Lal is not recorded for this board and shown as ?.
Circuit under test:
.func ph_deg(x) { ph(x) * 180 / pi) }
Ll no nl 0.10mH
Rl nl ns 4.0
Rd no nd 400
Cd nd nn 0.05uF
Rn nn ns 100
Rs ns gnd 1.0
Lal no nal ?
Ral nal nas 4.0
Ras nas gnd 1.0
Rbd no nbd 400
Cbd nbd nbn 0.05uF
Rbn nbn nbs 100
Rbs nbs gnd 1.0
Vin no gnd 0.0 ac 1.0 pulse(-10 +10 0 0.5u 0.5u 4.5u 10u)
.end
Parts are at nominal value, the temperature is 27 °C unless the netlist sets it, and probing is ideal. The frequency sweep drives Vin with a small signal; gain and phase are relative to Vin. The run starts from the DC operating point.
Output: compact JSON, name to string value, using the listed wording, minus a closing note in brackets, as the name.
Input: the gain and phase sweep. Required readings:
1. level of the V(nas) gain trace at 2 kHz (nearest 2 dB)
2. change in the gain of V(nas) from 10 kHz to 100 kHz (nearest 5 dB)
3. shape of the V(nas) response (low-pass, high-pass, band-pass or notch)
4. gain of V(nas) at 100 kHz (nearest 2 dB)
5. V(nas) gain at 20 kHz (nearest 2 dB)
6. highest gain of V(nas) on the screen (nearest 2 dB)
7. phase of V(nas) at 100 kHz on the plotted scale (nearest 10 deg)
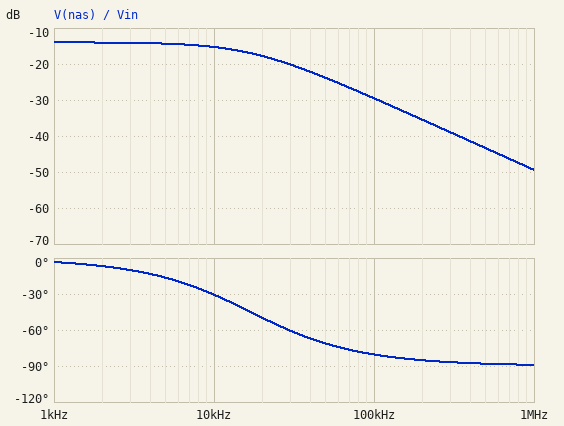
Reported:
{"level of the V(nas) gain trace at 2 kHz": "-14 dB", "change in the gain of V(nas) from 10 kHz to 100 kHz": "-15 dB", "shape of the V(nas) response": "low-pass", "gain of V(nas) at 100 kHz": "-30 dB", "V(nas) gain at 20 kHz": "-18 dB", "highest gain of V(nas) on the screen": "-14 dB", "phase of V(nas) at 100 kHz on the plotted scale": "-80 deg"}
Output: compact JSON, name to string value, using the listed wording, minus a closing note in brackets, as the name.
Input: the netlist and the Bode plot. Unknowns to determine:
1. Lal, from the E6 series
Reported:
{"Lal, from the E6 series": "47 µH"}
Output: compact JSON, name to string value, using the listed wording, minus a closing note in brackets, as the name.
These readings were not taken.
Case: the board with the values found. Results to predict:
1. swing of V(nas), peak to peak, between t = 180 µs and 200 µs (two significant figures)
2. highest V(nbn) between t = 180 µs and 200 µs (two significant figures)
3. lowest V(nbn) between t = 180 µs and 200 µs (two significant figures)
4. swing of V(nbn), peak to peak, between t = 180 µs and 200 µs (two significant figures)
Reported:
{"swing of V(nas), peak to peak, between t = 180 µs and 200 µs": "990 mV", "highest V(nbn) between t = 180 µs and 200 µs": "2.2 V", "lowest V(nbn) between t = 180 µs and 200 µs": "-2.2 V", "swing of V(nbn), peak to peak, between t = 180 µs and 200 µs": "4.4 V"}
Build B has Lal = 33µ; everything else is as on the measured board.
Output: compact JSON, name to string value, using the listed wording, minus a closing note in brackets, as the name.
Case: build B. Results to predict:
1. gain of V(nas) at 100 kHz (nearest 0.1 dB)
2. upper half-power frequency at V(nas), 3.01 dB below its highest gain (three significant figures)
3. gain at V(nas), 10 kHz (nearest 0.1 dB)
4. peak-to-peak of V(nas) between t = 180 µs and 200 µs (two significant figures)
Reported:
{"gain of V(nas) at 100 kHz": "-26.6 dB", "upper half-power frequency at V(nas), 3.01 dB below its highest gain": "24.1 kHz", "gain at V(nas), 10 kHz": "-14.7 dB", "peak-to-peak of V(nas) between t = 180 µs and 200 µs": "1.4 V"}
